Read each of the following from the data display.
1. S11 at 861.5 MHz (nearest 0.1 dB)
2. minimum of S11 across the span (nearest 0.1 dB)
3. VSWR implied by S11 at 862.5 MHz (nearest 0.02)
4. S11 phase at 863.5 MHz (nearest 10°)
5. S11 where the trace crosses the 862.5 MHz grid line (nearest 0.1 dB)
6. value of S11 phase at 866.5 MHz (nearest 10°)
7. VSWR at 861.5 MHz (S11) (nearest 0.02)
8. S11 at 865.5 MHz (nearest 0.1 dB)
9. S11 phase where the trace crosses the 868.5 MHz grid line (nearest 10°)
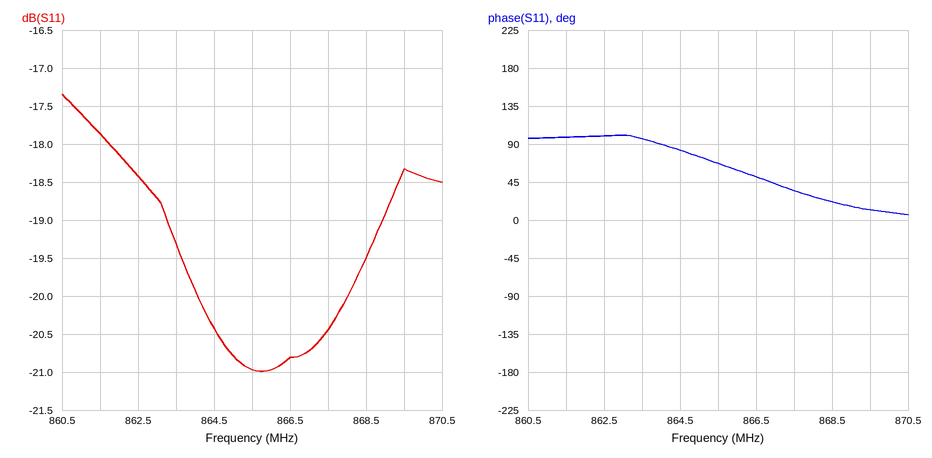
-17.9 dB
-21.0 dB
1.28
100°
-18.4 dB
50°
1.30
-21.0 dB
20°
